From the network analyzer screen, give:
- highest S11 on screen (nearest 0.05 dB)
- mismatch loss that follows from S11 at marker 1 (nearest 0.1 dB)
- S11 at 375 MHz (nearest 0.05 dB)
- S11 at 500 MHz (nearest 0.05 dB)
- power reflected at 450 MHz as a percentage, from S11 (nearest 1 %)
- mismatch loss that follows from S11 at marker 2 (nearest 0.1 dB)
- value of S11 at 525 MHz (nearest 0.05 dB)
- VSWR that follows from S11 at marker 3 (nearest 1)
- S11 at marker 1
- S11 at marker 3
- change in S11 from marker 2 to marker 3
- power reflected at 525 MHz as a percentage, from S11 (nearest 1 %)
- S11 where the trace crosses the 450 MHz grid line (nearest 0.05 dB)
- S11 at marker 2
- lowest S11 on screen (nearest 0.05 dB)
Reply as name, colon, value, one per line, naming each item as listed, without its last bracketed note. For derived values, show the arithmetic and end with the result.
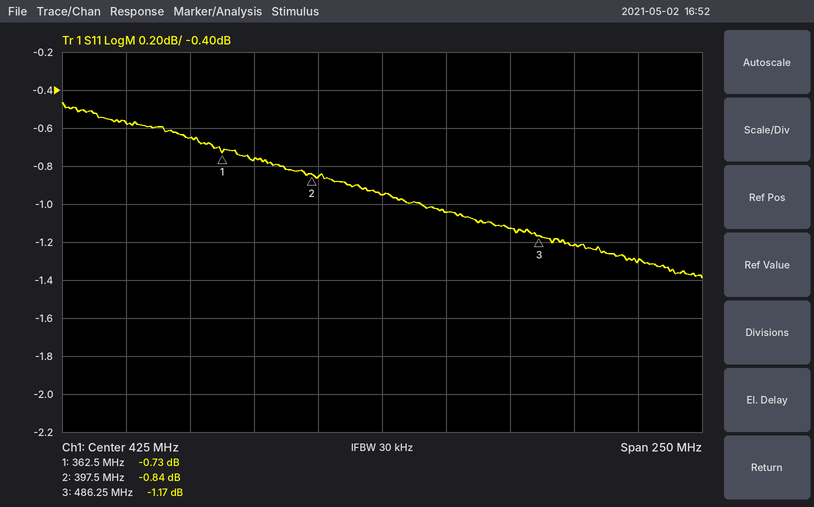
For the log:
highest S11 on screen: -0.45 dB
mismatch loss that follows from S11 at marker 1: −10 log10(1 − 10^(-0.73/10)) ≈ 8.1 dB
S11 at 375 MHz: -0.75 dB
S11 at 500 MHz: -1.20 dB
power reflected at 450 MHz as a percentage, from S11: 10^(-1.05/10) ≈ 79 %
mismatch loss that follows from S11 at marker 2: −10 log10(1 − 10^(-0.84/10)) ≈ 7.5 dB
value of S11 at 525 MHz: -1.30 dB
VSWR that follows from S11 at marker 3: (1 + 0.8740)/(1 − 0.8740) ≈ 15
S11 at marker 1: -0.73 dB
S11 at marker 3: -1.17 dB
change in S11 from marker 2 to marker 3: -1.17 − (-0.84) = -0.33 dB
power reflected at 525 MHz as a percentage, from S11: 10^(-1.3/10) ≈ 74 %
S11 where the trace crosses the 450 MHz grid line: -1.05 dB
S11 at marker 2: -0.84 dB
lowest S11 on screen: -1.40 dB
